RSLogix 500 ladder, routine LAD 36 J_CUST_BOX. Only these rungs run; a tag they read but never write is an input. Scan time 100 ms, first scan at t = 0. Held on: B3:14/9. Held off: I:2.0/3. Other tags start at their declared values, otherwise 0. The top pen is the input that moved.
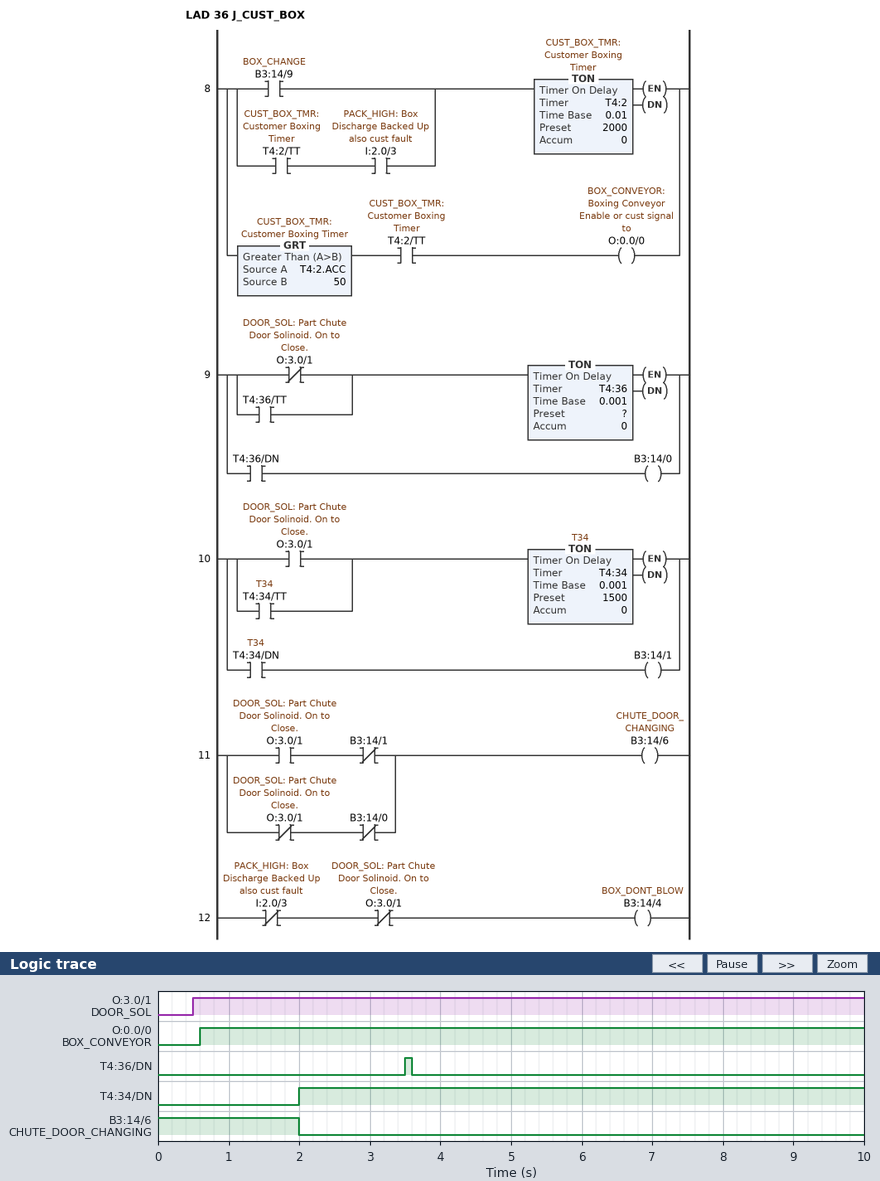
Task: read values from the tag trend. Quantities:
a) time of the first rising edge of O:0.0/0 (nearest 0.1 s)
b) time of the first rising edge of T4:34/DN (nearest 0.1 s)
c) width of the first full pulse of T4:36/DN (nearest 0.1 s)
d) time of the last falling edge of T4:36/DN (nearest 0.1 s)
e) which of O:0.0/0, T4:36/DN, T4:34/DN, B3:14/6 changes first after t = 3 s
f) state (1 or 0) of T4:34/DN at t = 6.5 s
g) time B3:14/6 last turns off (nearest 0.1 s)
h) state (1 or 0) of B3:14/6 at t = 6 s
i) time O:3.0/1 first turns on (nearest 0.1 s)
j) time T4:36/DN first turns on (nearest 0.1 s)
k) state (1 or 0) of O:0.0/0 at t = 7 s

0.6 s
2.0 s
0.1 s
3.6 s
T4:36/DN
1
2.0 s
0
0.5 s
3.5 s
1
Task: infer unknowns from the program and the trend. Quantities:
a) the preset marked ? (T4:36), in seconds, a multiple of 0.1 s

3.5 s
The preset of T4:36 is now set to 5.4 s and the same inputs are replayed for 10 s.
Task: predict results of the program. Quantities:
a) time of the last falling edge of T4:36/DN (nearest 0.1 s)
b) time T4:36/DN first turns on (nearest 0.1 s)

5.5 s
5.4 s
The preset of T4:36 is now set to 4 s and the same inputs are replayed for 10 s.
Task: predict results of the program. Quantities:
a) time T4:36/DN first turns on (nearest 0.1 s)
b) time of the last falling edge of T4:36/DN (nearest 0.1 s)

4.0 s
4.1 s
